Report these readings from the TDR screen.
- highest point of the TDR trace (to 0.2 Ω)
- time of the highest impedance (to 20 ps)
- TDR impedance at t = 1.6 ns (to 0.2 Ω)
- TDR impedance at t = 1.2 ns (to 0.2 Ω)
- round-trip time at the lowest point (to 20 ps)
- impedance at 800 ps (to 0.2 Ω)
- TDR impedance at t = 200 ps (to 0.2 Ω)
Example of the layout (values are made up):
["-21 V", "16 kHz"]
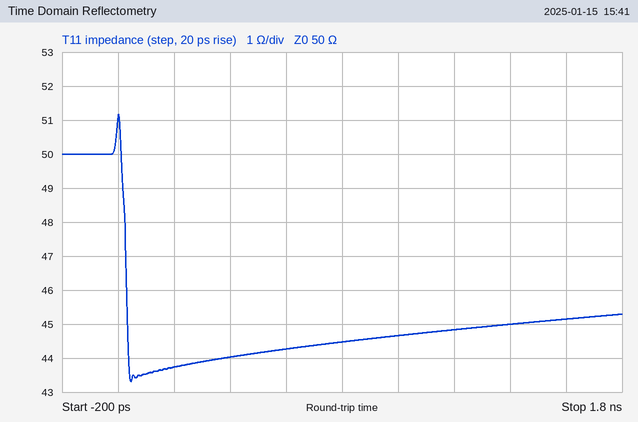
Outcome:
["51.2 Ω", "0 ps", "45.2 Ω", "44.8 Ω", "40 ps", "44.4 Ω", "43.8 Ω"]
